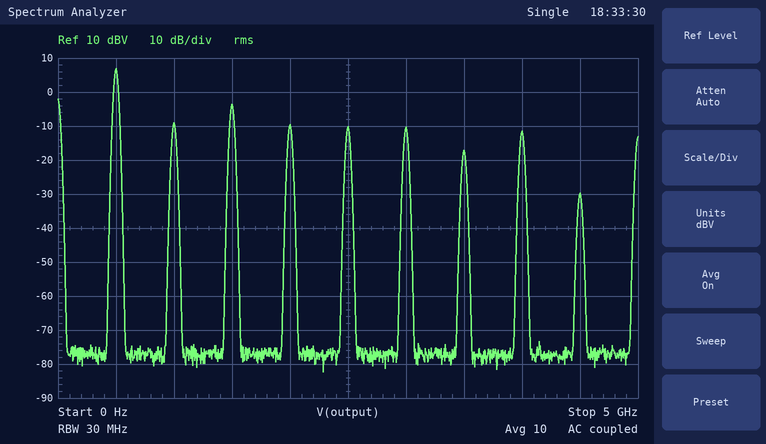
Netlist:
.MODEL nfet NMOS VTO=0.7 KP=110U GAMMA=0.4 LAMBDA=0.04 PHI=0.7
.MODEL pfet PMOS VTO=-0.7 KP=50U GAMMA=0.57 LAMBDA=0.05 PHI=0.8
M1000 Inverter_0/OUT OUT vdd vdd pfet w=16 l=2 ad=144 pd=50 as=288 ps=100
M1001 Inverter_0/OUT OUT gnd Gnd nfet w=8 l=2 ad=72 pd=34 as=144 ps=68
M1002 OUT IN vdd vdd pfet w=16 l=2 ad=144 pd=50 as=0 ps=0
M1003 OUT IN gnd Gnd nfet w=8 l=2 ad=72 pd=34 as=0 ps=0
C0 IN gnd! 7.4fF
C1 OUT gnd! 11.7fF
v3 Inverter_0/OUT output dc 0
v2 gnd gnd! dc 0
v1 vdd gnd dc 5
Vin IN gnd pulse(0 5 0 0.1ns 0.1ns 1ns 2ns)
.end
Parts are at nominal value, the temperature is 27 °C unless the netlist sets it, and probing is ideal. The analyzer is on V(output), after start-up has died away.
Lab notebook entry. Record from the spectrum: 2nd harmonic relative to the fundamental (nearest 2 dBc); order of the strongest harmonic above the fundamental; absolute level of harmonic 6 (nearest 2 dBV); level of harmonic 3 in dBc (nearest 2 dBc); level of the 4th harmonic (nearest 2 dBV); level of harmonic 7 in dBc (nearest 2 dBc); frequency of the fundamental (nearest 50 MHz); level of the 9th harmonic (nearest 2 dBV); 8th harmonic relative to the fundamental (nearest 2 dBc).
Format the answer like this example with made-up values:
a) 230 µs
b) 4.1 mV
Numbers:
a) -16 dBc
b) 3
c) -10 dBV
d) -10 dBc
e) -10 dBV
f) -24 dBc
g) 500 MHz
h) -30 dBV
i) -18 dBc
